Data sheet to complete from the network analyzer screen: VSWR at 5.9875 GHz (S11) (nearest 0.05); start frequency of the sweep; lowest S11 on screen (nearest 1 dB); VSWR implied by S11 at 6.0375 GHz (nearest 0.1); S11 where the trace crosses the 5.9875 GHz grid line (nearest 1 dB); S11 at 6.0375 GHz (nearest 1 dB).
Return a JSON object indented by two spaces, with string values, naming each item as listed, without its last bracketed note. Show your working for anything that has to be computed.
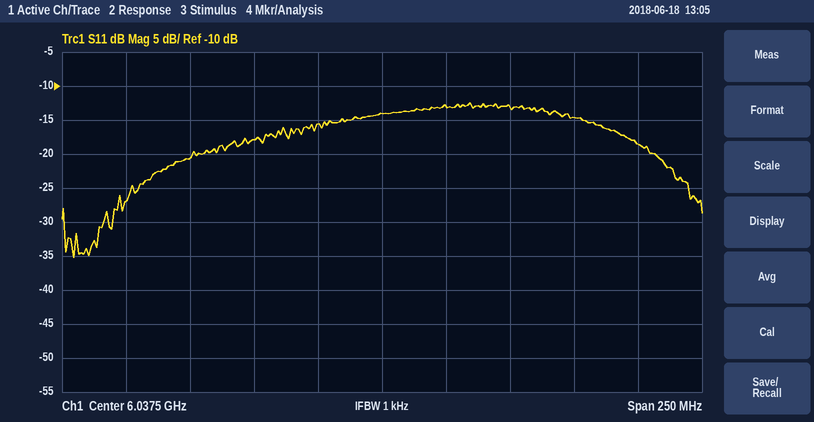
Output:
{
  "VSWR at 5.9875 GHz (S11)": "|Γ| = 10^(-18/20) = 0.1259; VSWR = (1 + 0.1259)/(1 − 0.1259) ≈ 1.29, so 1.30 to the nearest 0.05",
  "start frequency of the sweep": "5.9125 GHz",
  "lowest S11 on screen": "-35 dB",
  "VSWR implied by S11 at 6.0375 GHz": "|Γ| = 10^(-14/20) = 0.1995; VSWR = (1 + 0.1995)/(1 − 0.1995) ≈ 1.5",
  "S11 where the trace crosses the 5.9875 GHz grid line": "-18 dB",
  "S11 at 6.0375 GHz": "-14 dB"
}
